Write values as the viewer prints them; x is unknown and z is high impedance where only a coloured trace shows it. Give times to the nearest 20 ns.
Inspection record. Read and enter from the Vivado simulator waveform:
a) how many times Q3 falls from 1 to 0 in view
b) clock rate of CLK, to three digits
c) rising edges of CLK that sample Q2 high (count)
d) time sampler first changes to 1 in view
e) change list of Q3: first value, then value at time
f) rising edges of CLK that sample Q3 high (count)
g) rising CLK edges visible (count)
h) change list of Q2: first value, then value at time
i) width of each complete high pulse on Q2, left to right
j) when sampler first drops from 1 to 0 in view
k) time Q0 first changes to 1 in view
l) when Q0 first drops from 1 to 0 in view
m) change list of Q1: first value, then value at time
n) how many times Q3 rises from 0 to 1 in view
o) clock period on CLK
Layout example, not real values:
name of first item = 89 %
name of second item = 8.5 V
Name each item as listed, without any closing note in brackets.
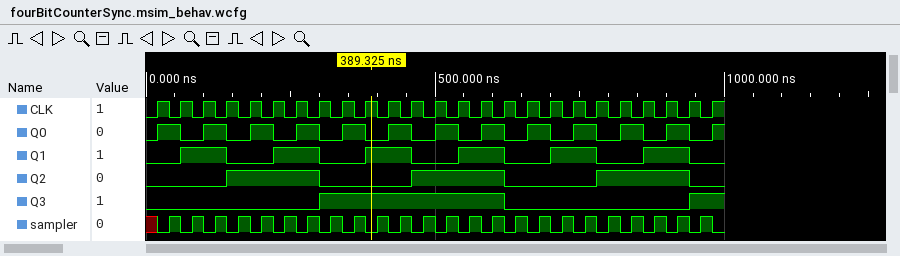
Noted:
how many times Q3 falls from 1 to 0 in view = 1
clock rate of CLK, to three digits = 25.0 MHz
rising edges of CLK that sample Q2 high = 12
time sampler first changes to 1 in view = 40 ns
change list of Q3: first value, then value at time = 0, 1 at 300 ns, 0 at 620 ns, 1 at 940 ns
rising edges of CLK that sample Q3 high = 9
rising CLK edges visible = 25
change list of Q2: first value, then value at time = 0, 1 at 140 ns, 0 at 300 ns, 1 at 460 ns, 0 at 620 ns, 1 at 780 ns, 0 at 940 ns
width of each complete high pulse on Q2, left to right = 160 ns, 160 ns, 160 ns
when sampler first drops from 1 to 0 in view = 60 ns
time Q0 first changes to 1 in view = 20 ns
when Q0 first drops from 1 to 0 in view = 60 ns
change list of Q1: first value, then value at time = 0, 1 at 60 ns, 0 at 140 ns, 1 at 220 ns, 0 at 300 ns, 1 at 380 ns, 0 at 460 ns, 1 at 540 ns, 0 at 620 ns, 1 at 700 ns, 0 at 780 ns, 1 at 860 ns, 0 at 940 ns
how many times Q3 rises from 0 to 1 in view = 2
clock period on CLK = 40 ns
